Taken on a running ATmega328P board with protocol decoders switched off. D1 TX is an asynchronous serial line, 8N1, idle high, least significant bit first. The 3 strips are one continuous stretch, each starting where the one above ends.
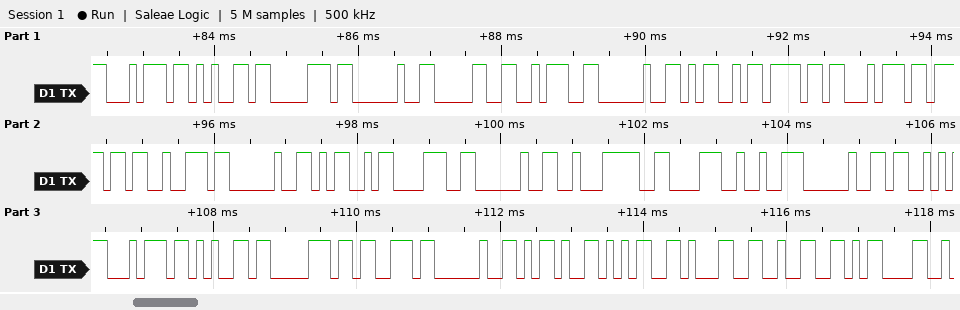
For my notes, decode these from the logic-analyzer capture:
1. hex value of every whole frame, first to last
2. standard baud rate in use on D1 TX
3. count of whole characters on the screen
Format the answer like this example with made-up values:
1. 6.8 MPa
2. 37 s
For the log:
1. 74 65 70 20 30 3A 20 4D 6F 74 6F 72 20 4D 38 20 E2 86 92 20 53 74 65 70 73 20 2D 35 31 32 0D
2. 9600 baud
3. 31
